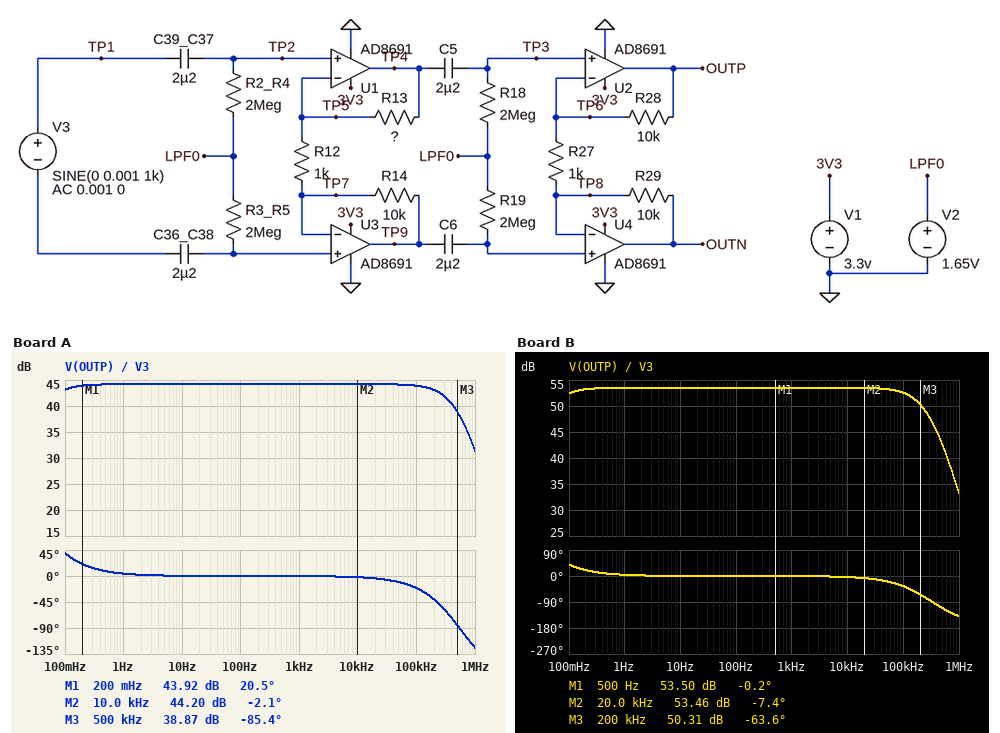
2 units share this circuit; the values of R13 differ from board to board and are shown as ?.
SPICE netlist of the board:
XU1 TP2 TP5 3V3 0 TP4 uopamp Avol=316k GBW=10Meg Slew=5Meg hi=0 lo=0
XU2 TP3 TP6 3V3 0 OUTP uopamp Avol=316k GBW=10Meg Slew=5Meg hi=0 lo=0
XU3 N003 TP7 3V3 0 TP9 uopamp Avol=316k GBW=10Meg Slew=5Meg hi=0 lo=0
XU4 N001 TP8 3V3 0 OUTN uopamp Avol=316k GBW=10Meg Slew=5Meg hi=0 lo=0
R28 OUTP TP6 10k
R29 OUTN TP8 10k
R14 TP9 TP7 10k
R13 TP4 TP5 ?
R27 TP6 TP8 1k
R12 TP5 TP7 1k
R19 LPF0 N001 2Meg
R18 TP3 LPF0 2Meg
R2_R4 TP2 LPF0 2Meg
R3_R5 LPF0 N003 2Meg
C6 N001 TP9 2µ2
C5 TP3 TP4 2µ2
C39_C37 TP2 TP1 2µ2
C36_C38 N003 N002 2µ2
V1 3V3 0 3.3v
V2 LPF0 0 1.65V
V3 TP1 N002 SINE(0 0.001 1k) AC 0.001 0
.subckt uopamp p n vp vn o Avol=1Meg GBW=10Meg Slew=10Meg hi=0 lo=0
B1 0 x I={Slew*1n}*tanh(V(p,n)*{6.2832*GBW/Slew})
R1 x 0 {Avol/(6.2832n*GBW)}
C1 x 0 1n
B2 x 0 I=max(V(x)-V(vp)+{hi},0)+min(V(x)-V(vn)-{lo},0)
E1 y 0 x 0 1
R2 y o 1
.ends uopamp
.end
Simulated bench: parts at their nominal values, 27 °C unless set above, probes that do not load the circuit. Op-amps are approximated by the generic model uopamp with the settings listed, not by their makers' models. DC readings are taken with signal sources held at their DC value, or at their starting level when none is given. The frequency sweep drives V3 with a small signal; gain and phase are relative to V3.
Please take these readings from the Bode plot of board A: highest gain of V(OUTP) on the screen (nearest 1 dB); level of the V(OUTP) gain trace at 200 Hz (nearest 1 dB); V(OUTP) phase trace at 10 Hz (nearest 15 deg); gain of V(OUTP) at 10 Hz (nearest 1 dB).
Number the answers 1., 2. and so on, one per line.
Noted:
1. 44 dB
2. 44 dB
3. 0 deg
4. 44 dB
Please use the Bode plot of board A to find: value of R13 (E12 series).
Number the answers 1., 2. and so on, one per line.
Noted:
1. 4.7 kΩ
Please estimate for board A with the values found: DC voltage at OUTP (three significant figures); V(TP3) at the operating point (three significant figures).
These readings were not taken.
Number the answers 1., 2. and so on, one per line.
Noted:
1. 1.65 V
2. 1.65 V
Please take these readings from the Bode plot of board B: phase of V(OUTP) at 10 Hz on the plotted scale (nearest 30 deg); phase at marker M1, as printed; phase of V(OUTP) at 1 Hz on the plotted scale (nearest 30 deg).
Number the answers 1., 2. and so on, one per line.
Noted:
1. 0 deg
2. -0.2 deg
3. 0 deg
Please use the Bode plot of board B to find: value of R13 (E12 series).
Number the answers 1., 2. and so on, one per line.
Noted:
1. 33 kΩ
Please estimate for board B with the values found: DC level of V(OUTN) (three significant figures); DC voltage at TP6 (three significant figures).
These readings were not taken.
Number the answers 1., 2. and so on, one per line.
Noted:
1. 1.65 V
2. 1.65 V
